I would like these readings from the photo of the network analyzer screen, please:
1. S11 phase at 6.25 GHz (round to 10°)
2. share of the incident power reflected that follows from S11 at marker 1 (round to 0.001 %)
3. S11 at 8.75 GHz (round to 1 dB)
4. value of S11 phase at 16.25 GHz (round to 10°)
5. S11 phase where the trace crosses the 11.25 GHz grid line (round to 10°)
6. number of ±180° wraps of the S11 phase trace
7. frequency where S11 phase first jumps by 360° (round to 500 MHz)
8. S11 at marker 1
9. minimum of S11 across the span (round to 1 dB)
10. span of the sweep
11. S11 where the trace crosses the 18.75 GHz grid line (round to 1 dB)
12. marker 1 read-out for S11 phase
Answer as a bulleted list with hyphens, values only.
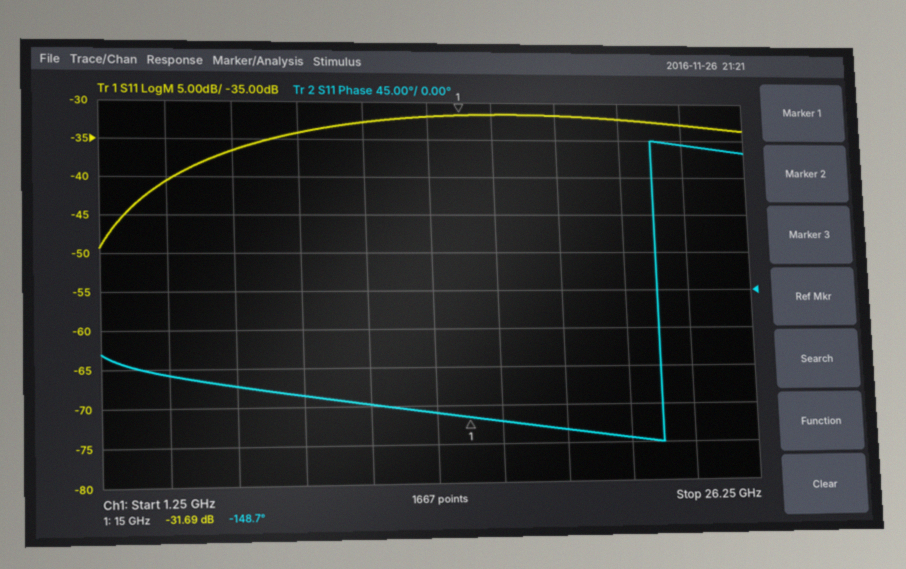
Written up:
- -110°
- 0.068 %
- -34 dB
- -150°
- -130°
- 1
- 22.5 GHz
- -31.69 dB
- -49 dB
- 25 GHz
- -32 dB
- -148.7°
